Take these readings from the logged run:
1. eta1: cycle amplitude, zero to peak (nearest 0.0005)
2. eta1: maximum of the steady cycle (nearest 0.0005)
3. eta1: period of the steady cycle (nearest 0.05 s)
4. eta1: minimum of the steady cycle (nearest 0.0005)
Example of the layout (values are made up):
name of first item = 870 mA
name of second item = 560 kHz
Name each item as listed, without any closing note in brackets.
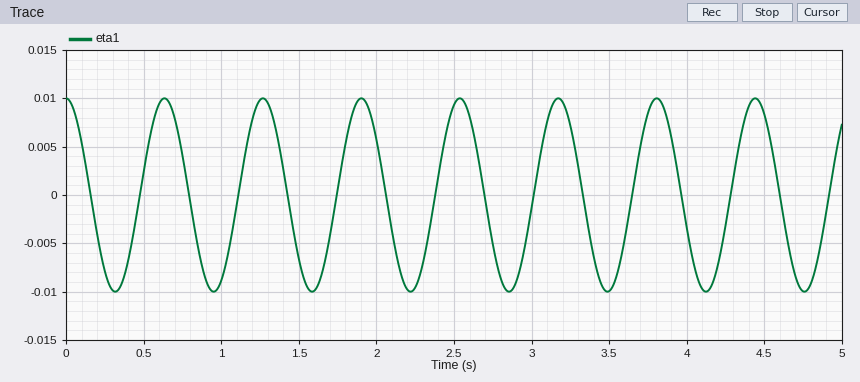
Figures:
eta1: cycle amplitude, zero to peak = 0.0100
eta1: maximum of the steady cycle = 0.0100
eta1: period of the steady cycle = 0.65 s
eta1: minimum of the steady cycle = -0.0100
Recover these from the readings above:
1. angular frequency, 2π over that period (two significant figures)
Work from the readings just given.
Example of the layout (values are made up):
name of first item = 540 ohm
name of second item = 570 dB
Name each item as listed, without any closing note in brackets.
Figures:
angular frequency, 2π over that period = 9.7 rad/s
